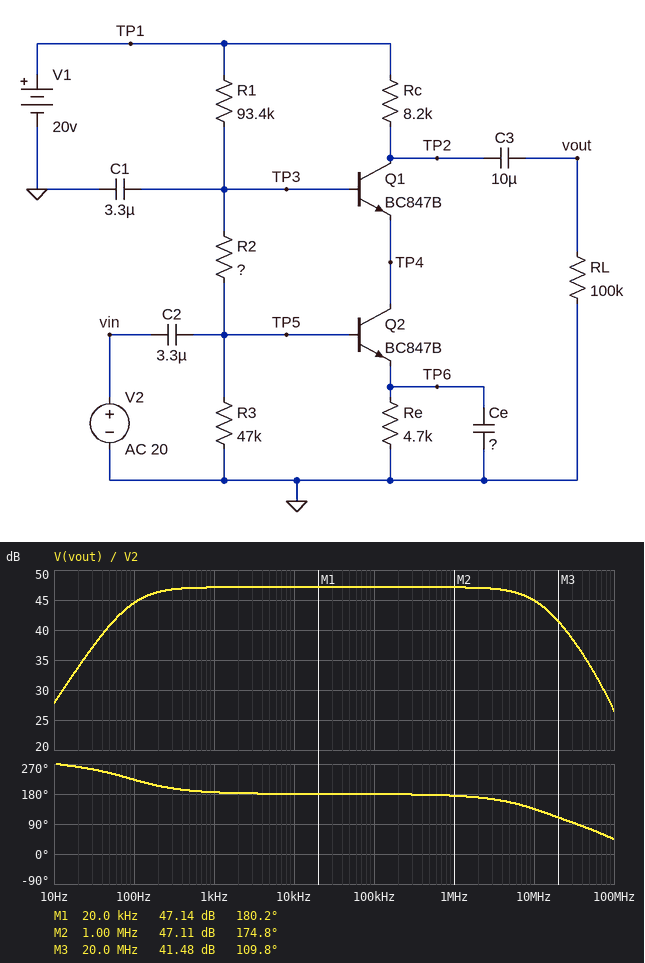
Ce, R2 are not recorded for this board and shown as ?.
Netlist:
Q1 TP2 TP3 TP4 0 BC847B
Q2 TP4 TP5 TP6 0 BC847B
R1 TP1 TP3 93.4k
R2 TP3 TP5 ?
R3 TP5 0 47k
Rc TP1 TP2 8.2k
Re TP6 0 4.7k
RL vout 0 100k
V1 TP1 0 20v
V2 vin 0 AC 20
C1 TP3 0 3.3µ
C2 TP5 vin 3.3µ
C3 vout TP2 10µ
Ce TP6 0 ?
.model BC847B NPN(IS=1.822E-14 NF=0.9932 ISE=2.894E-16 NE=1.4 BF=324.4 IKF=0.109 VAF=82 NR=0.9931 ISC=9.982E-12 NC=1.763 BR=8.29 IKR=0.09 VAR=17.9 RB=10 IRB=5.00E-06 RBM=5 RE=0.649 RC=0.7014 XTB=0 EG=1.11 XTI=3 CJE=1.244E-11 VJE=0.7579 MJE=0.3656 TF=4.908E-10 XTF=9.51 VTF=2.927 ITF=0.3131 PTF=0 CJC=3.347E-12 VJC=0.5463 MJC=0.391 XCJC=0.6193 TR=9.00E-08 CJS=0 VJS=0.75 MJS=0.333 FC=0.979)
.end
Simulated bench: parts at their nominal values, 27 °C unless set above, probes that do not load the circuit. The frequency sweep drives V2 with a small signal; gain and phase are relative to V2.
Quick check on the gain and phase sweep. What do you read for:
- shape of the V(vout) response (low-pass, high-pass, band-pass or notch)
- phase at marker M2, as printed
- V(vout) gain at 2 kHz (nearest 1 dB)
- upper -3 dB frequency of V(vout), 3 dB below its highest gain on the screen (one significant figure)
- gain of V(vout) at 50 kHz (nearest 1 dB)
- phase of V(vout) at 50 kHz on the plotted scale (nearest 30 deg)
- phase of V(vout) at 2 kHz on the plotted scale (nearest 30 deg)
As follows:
band-pass
174.8 deg
47 dB
10 MHz
47 dB
180 deg
180 deg
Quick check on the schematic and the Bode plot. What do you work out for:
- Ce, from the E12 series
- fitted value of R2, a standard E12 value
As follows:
56 µF
68 kΩ
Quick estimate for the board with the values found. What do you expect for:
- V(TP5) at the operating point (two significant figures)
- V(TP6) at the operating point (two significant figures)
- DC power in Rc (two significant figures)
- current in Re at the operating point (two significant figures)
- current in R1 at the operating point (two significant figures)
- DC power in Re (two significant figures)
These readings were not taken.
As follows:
4.4 V
3.7 V
5.1 mW
800 µA
98 µA
3.0 mW
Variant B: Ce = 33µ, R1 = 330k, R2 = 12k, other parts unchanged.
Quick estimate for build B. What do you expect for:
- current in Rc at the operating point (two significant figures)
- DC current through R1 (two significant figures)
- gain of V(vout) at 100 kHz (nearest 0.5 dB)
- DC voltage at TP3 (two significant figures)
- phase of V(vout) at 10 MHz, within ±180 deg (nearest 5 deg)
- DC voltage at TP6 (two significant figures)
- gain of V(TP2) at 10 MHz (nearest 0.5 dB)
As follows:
360 µA
52 µA
40.5 dB
2.9 V
145 deg
1.7 V
39.5 dB
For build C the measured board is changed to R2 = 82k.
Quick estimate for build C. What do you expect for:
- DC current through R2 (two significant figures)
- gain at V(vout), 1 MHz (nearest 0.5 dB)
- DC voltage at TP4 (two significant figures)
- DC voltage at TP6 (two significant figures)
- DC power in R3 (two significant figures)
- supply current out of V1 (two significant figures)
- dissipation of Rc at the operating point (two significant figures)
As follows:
89 µA
46.5 dB
11 V
3.5 V
360 µW
830 µA
4.4 mW
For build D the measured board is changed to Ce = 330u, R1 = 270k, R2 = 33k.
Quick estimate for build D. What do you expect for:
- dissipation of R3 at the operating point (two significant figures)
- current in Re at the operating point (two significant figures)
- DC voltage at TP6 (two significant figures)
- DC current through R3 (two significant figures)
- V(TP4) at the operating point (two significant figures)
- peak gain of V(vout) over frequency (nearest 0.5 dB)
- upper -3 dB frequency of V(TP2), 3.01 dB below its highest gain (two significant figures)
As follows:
140 µW
420 µA
2.0 V
55 µA
3.8 V
41.5 dB
20 MHz
